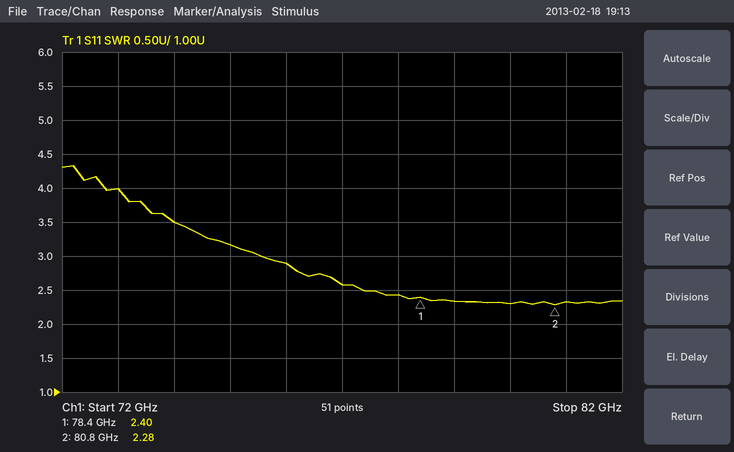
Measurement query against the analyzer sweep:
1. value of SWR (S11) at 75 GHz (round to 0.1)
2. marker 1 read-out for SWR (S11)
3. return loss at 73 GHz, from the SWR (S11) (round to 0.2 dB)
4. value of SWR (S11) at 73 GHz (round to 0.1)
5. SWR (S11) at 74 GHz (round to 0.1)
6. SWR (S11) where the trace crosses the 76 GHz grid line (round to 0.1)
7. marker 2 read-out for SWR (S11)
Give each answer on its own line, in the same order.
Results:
3.2
2.40
4.4 dB
4.0
3.5
2.9
2.28
